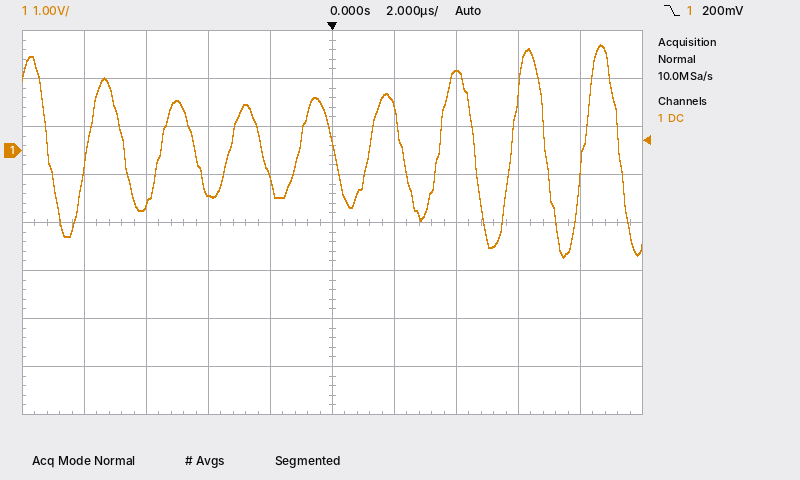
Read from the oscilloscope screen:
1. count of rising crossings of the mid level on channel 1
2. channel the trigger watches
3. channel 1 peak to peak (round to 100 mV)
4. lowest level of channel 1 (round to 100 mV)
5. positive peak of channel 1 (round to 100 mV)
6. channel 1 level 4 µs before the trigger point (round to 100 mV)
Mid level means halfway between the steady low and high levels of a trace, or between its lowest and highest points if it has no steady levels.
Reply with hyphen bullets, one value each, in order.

- 8
- channel 1
- 4.4 V
- -2.2 V
- 2.2 V
- -900 mV
